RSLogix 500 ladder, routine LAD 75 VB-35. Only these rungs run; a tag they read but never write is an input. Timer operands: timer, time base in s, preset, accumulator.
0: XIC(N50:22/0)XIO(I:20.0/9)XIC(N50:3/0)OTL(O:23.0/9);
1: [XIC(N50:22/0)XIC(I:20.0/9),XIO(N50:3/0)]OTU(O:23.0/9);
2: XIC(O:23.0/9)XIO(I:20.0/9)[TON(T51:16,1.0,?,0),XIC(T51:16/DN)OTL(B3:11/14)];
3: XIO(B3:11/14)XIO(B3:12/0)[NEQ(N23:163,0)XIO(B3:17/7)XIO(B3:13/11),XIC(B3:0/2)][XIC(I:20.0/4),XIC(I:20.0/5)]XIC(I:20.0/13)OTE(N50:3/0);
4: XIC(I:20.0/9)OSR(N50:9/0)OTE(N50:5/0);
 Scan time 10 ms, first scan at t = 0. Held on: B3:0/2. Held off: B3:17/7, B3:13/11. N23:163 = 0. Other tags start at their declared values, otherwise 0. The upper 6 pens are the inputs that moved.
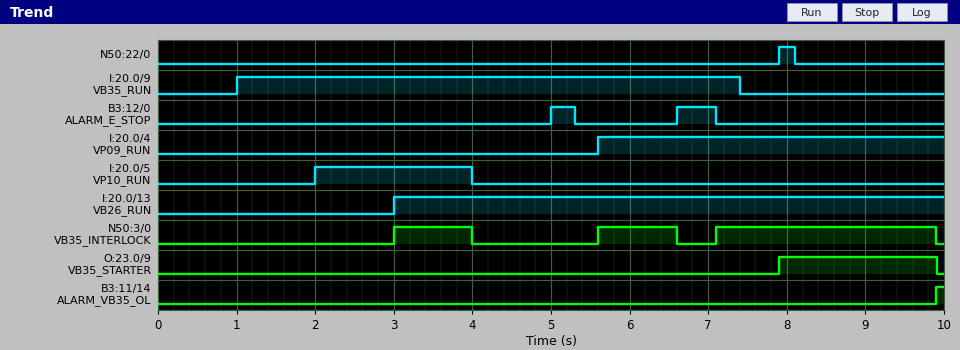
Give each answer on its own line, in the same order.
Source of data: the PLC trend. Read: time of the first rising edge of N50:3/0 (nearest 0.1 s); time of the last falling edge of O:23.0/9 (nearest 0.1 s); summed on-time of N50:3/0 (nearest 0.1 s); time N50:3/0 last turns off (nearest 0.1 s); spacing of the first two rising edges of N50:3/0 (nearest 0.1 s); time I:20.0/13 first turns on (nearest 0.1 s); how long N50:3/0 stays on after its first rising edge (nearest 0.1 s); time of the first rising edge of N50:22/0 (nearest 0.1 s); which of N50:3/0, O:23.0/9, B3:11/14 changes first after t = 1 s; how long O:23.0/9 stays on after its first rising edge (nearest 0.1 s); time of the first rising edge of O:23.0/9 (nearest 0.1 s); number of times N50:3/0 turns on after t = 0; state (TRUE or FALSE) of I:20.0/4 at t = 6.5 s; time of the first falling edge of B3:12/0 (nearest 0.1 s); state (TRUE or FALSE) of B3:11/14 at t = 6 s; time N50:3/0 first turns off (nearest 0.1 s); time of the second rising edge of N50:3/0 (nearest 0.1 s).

3.0 s
9.9 s
4.8 s
9.9 s
2.6 s
3.0 s
1.0 s
7.9 s
N50:3/0
2.0 s
7.9 s
3
TRUE
5.3 s
FALSE
4.0 s
5.6 s
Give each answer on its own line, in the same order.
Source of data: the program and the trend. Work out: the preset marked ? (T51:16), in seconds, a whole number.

2 s
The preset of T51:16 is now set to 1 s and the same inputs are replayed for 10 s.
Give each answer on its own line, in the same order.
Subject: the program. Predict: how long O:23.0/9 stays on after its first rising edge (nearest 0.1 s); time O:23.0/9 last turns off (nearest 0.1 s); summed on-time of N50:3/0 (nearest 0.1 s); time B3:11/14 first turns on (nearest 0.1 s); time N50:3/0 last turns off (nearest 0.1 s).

1.0 s
8.9 s
3.8 s
8.9 s
8.9 s
